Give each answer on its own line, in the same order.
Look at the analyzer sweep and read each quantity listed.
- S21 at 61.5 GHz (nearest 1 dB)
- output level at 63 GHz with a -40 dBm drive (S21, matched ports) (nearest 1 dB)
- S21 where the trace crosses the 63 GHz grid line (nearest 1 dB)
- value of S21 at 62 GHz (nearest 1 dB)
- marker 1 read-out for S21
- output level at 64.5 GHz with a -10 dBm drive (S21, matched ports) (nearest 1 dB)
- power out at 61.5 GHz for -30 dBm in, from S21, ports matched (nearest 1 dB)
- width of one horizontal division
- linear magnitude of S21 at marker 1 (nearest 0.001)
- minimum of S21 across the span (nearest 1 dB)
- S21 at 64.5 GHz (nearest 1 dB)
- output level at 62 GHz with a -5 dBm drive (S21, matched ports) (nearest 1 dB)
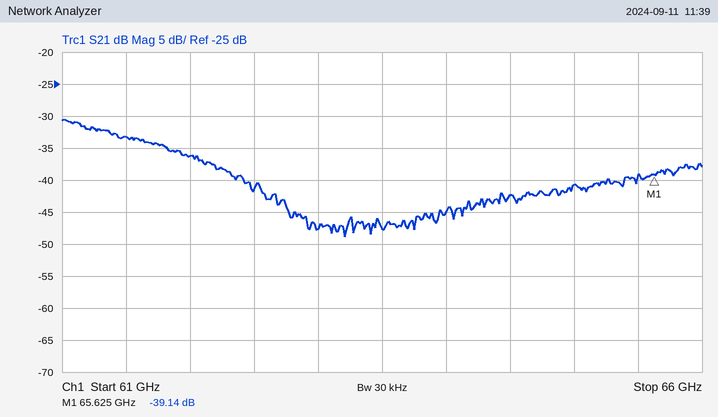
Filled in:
-33 dB
-88 dBm
-48 dB
-36 dB
-39.14 dB
-52 dBm
-63 dBm
500 MHz
0.011
-49 dB
-42 dB
-41 dBm
